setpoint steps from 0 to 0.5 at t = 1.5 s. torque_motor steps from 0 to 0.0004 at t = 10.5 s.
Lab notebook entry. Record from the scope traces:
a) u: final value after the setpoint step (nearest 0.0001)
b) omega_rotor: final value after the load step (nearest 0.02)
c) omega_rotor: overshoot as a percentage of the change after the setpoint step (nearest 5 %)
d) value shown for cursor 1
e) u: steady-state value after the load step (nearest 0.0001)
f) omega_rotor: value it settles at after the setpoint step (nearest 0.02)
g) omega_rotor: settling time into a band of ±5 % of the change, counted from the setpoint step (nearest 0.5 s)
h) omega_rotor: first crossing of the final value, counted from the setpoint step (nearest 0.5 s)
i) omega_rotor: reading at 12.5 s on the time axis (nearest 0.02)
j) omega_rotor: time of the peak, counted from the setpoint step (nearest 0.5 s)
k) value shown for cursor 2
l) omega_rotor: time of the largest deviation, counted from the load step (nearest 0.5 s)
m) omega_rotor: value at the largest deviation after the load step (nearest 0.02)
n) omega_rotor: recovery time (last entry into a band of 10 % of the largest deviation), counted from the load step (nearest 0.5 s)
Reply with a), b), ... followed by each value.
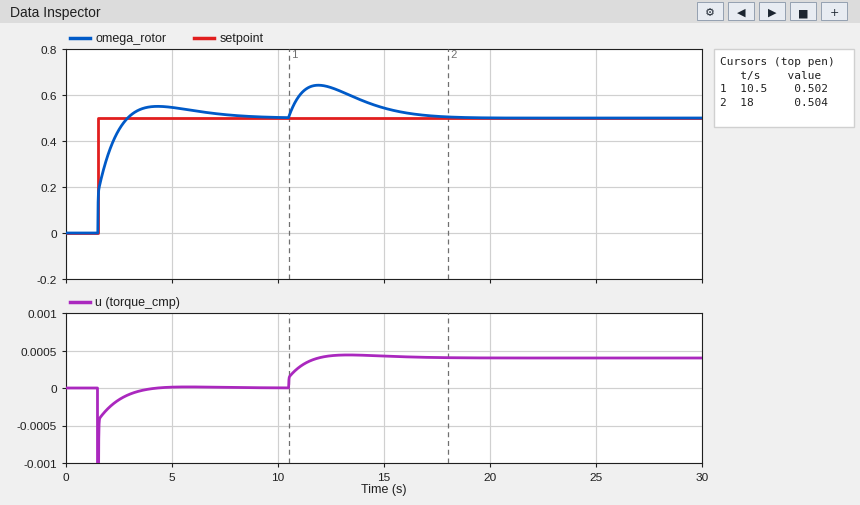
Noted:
a) 0.0000
b) 0.50
c) 10 %
d) 0.502
e) 0.0004
f) 0.50
g) 5.0 s
h) 1.5 s
i) 0.64
j) 3.0 s
k) 0.504
l) 1.5 s
m) 0.64
n) 6.0 s
